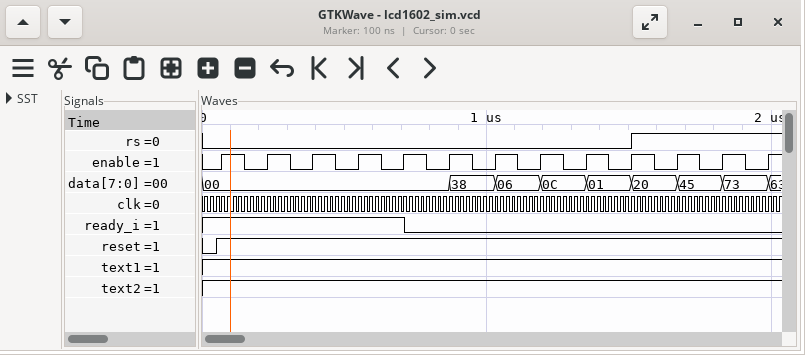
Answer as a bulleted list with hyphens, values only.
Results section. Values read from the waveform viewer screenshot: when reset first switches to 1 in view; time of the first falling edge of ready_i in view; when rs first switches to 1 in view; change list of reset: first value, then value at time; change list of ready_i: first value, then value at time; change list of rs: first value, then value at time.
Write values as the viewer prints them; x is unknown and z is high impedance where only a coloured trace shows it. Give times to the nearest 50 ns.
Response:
- 50 ns
- 700 ns
- 1500 ns
- 0, 1 at 50 ns
- 1, 0 at 700 ns
- 0, 1 at 1500 ns
